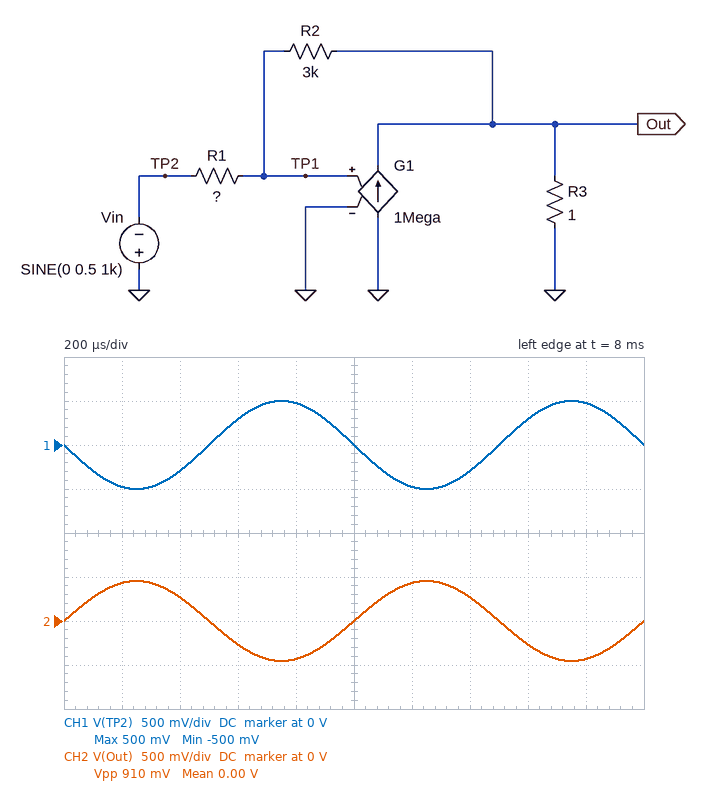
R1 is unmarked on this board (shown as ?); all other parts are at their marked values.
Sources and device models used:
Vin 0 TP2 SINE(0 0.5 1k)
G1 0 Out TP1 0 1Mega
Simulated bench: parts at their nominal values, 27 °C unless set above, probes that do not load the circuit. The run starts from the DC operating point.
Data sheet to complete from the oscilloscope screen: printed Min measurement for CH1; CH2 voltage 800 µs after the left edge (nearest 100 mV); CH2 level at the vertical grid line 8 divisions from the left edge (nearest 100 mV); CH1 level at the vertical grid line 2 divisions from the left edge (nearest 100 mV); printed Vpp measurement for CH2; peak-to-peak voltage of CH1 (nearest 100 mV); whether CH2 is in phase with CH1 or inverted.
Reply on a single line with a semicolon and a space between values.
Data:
-500 mV; -400 mV; -300 mV; -300 mV; 910 mV; 1.0 V; inverted
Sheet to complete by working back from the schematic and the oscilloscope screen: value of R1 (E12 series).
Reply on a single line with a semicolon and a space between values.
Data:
3.3 kΩ
